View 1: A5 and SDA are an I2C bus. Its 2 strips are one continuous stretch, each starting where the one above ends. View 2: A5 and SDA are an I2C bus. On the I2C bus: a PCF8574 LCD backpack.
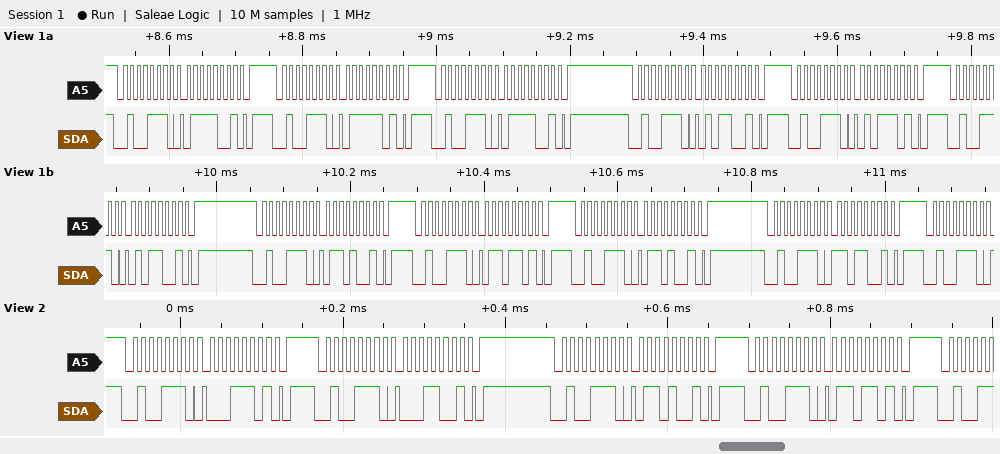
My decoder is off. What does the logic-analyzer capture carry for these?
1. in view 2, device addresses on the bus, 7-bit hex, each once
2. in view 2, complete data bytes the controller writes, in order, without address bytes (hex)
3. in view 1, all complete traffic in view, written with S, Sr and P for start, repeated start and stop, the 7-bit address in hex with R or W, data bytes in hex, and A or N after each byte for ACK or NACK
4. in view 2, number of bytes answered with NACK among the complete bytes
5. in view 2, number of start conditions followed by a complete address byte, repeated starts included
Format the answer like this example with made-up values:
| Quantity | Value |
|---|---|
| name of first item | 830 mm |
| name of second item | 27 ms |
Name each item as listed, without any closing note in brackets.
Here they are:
| Quantity | Value |
|---|---|
| in view 2, device addresses on the bus, 7-bit hex, each once | 0x27 |
| in view 2, complete data bytes the controller writes, in order, without address bytes | 1D 19 69 6D |
| in view 1, all complete traffic in view, written with S, Sr and P for start, repeated start and stop, the 7-bit address in hex with R or W, data bytes in hex, and A or N after each byte for ACK or NACK | S 27W A 79 A P S 27W A 7D A P S 27W A 79 A P S 27W A 59 A P S 27W A 5D A P S 27W A 59 A P S 27W A 69 A P S 27W A 6D A P S 27W A 69 A P S 27W A D9 A P S 27W A |
| in view 2, number of bytes answered with NACK among the complete bytes | 0 |
| in view 2, number of start conditions followed by a complete address byte, repeated starts included | 4 |
